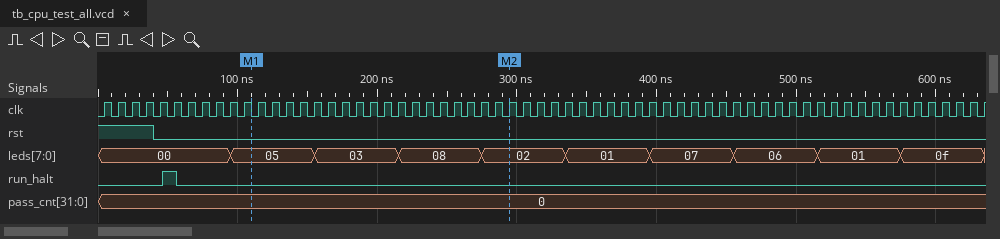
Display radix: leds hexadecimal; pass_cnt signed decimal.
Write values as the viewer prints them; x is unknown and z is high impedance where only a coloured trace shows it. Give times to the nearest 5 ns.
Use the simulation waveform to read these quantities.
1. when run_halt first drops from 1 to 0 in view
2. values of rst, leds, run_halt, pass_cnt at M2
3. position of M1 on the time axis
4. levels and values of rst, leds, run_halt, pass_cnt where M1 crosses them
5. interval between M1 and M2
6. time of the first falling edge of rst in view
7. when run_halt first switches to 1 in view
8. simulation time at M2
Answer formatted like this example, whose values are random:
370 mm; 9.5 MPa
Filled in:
55 ns; rst=0, leds=02, run_halt=0, pass_cnt=0; 110 ns; rst=0, leds=05, run_halt=0, pass_cnt=0; 185 ns; 40 ns; 45 ns; 295 ns
